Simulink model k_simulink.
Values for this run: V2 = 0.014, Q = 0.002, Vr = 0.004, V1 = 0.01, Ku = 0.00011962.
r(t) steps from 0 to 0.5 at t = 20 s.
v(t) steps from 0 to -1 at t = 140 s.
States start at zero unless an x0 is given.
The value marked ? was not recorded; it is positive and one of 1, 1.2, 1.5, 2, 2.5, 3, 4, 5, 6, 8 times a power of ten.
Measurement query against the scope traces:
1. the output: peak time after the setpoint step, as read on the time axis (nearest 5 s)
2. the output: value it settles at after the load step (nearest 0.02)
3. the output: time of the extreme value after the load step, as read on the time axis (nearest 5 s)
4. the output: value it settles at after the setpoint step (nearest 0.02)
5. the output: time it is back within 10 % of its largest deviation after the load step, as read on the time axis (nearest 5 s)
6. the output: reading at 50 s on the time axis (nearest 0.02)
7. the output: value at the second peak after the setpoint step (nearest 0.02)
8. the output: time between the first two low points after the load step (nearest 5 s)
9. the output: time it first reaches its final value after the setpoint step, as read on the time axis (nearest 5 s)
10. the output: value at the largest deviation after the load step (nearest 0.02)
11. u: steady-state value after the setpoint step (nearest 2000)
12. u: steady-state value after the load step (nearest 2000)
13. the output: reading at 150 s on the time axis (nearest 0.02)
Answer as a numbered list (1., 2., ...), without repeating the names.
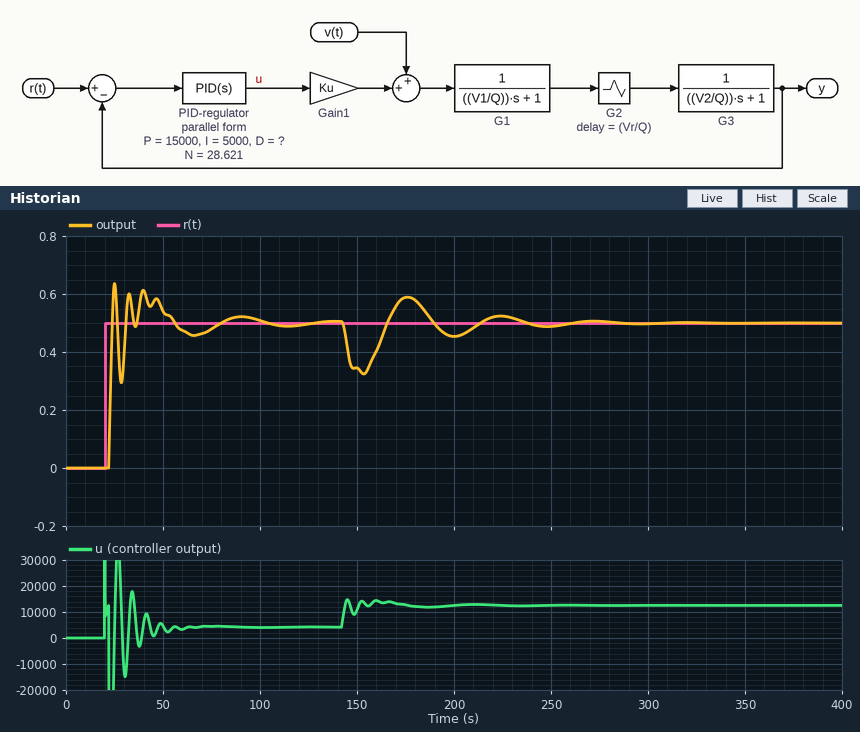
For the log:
1. 25 s
2. 0.50
3. 155 s
4. 0.50
5. 230 s
6. 0.54
7. 0.60
8. 45 s
9. 25 s
10. 0.32
11. 4000
12. 12000
13. 0.34
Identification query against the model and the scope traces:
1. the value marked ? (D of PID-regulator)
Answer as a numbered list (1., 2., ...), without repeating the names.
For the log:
1. 200000
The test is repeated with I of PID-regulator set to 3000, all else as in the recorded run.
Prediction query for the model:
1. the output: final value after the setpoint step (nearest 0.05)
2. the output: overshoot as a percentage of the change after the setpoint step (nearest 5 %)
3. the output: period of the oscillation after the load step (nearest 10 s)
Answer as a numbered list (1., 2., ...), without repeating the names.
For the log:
1. 0.50
2. 25 %
3. 60 s
